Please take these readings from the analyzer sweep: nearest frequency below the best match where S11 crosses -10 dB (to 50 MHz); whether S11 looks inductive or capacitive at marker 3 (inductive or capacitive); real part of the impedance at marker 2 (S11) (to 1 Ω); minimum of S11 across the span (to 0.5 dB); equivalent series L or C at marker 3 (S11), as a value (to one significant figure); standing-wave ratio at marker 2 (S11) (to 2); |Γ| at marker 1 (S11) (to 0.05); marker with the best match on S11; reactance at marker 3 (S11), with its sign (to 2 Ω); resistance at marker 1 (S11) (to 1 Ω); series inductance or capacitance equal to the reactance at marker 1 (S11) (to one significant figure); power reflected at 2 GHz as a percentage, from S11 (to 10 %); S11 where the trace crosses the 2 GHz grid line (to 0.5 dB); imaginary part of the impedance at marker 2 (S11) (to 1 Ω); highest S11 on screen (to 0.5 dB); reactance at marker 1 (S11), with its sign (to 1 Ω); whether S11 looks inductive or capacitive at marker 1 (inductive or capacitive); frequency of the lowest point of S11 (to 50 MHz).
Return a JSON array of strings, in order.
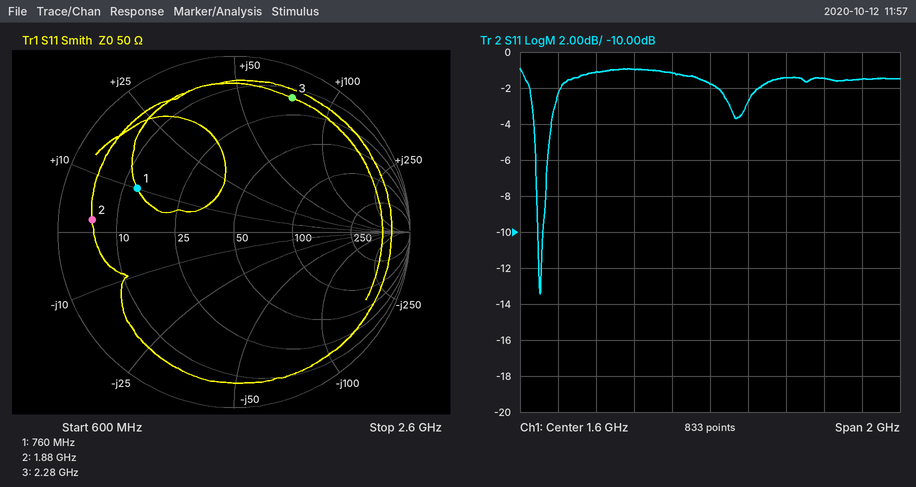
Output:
["700 MHz", "inductive", "5 Ω", "-13.5 dB", "5 nH", "10", "0.60", "marker 1", "+74 Ω", "13 Ω", "2 nH", "70 %", "-1.5 dB", "+2 Ω", "-1.0 dB", "+10 Ω", "inductive", "700 MHz"]
